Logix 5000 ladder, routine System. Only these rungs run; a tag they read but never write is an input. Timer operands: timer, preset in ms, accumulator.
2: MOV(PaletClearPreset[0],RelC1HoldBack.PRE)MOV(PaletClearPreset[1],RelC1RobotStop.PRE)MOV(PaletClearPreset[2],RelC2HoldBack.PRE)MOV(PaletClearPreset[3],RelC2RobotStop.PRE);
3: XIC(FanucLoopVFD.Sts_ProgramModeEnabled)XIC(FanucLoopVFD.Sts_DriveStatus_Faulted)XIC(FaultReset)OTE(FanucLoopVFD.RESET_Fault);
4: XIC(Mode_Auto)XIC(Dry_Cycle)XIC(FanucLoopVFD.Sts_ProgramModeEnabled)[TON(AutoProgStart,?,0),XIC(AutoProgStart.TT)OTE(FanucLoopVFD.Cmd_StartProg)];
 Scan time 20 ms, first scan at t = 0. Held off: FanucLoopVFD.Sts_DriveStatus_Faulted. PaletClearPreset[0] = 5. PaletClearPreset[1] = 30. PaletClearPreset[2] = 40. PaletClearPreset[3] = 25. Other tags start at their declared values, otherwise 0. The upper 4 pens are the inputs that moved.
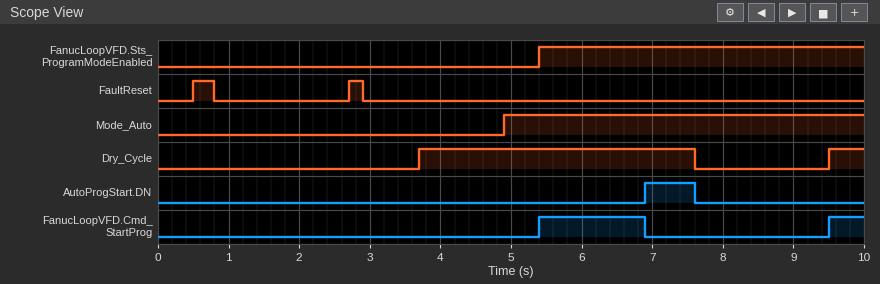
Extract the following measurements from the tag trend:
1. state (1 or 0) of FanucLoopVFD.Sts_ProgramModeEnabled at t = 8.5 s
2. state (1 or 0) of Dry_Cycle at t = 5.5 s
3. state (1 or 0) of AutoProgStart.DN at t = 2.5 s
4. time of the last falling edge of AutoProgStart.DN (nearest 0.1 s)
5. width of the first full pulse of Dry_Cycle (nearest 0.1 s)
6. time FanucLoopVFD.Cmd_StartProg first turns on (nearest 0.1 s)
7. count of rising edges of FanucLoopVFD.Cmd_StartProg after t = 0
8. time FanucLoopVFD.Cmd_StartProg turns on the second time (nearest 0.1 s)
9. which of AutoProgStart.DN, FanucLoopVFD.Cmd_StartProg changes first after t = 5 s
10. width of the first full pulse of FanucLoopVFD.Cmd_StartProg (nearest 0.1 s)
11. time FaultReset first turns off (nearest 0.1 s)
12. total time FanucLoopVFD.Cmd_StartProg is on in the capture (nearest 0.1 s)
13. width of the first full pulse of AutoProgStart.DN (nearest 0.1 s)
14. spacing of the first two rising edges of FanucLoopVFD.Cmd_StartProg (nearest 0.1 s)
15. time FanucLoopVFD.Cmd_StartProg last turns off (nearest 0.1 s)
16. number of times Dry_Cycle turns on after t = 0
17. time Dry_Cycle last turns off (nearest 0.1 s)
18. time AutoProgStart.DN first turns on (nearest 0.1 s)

1
1
0
7.6 s
3.9 s
5.4 s
2
9.5 s
FanucLoopVFD.Cmd_StartProg
1.5 s
0.8 s
2.0 s
0.7 s
4.1 s
6.9 s
2
7.6 s
6.9 s
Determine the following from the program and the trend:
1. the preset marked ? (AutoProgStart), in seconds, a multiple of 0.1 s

1.5 s
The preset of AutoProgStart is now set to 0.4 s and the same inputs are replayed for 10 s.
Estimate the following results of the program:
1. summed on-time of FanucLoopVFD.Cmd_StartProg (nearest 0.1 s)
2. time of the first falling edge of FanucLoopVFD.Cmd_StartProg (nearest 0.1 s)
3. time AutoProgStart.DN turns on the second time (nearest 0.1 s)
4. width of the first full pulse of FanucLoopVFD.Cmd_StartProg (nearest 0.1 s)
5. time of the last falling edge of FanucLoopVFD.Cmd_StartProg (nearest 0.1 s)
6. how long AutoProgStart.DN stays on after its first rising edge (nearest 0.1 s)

0.8 s
5.8 s
9.9 s
0.4 s
9.9 s
1.8 s
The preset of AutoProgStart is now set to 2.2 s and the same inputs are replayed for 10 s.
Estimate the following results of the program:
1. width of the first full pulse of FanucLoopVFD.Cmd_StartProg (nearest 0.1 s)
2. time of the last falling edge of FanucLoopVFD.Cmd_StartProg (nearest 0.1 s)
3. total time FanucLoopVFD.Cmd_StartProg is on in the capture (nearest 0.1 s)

2.2 s
7.6 s
2.7 s
